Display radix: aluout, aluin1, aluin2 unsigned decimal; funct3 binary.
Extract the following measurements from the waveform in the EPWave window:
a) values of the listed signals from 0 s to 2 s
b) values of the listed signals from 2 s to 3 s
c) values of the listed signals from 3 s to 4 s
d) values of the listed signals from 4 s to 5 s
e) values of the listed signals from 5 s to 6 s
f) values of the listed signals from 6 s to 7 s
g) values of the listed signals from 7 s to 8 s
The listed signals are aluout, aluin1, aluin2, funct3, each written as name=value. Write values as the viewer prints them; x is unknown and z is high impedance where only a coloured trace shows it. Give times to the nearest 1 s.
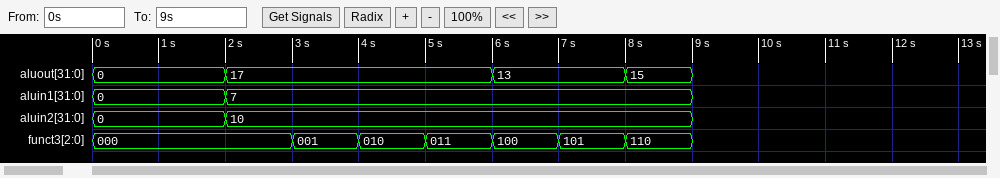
aluout=0, aluin1=0, aluin2=0, funct3=000
aluout=17, aluin1=7, aluin2=10, funct3=000
aluout=17, aluin1=7, aluin2=10, funct3=001
aluout=17, aluin1=7, aluin2=10, funct3=010
aluout=17, aluin1=7, aluin2=10, funct3=011
aluout=13, aluin1=7, aluin2=10, funct3=100
aluout=13, aluin1=7, aluin2=10, funct3=101
